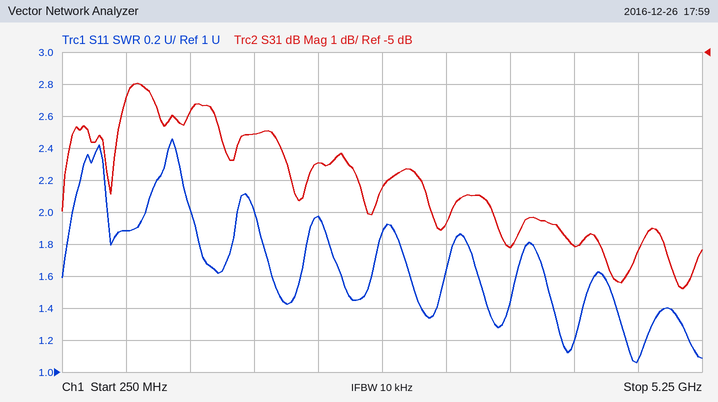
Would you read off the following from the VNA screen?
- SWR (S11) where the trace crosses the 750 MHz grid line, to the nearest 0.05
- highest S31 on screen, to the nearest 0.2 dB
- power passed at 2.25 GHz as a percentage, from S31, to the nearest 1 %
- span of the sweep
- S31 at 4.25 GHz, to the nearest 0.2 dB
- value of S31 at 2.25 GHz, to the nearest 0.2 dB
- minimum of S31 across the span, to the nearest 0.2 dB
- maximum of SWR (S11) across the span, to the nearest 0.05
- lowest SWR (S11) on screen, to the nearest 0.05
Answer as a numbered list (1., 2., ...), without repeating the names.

1. 1.90
2. -6.0 dB
3. 14 %
4. 5 GHz
5. -11.0 dB
6. -8.4 dB
7. -12.4 dB
8. 2.45
9. 1.05
